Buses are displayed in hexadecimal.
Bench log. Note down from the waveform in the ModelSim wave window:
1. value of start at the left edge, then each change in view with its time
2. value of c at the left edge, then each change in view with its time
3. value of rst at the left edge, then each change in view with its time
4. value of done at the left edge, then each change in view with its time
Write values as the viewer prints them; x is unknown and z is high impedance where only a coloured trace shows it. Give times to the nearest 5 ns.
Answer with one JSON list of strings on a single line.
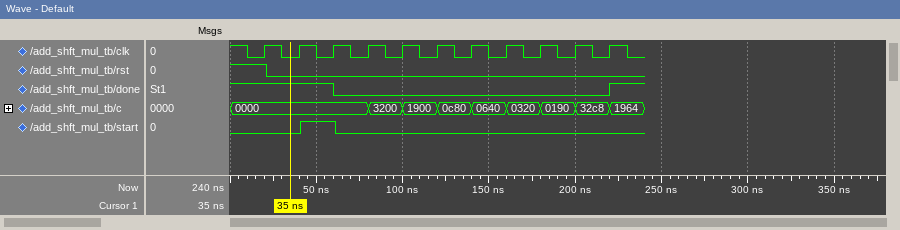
["0, 1 at 40 ns, 0 at 60 ns", "0000, 3200 at 80 ns, 1900 at 100 ns, 0c80 at 120 ns, 0640 at 140 ns, 0320 at 160 ns, 0190 at 180 ns, 32c8 at 200 ns, 1964 at 220 ns", "1, 0 at 20 ns", "1, 0 at 60 ns, 1 at 220 ns"]
